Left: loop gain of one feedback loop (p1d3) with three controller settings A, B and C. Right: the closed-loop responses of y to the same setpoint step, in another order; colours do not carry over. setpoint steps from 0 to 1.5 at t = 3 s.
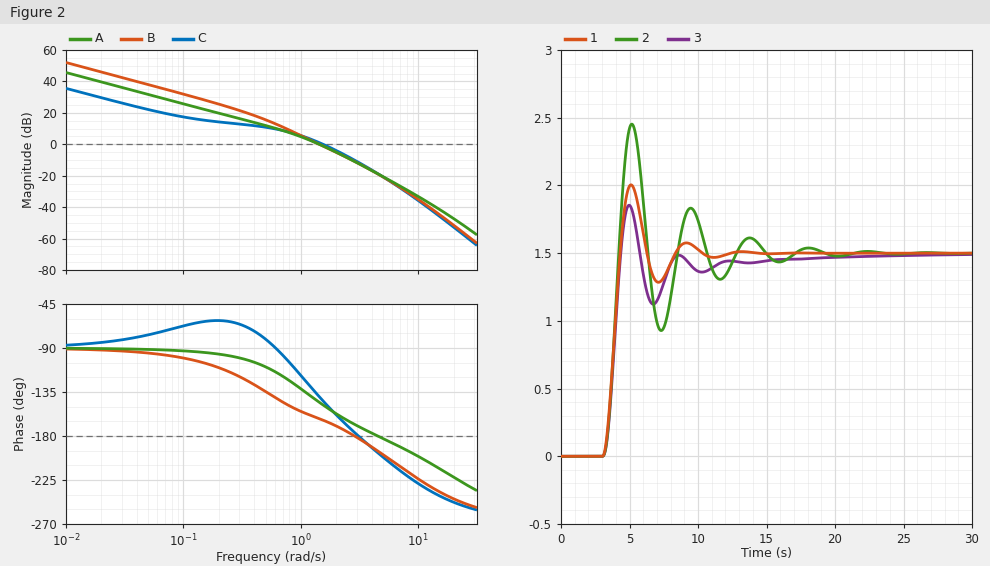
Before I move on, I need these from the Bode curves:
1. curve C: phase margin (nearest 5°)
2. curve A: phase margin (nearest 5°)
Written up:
35°
35°
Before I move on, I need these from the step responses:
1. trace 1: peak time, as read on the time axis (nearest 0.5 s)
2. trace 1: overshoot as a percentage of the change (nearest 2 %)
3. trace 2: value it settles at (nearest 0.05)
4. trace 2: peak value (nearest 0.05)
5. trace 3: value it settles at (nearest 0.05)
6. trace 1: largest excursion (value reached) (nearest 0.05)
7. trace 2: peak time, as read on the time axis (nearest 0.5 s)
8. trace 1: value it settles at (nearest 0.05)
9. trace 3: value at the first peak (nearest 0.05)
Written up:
5.0 s
34 %
1.50
2.45
1.50
2.00
5.0 s
1.50
1.85
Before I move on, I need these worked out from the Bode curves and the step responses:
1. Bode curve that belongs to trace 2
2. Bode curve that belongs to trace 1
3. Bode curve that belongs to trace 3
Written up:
B
A
C
